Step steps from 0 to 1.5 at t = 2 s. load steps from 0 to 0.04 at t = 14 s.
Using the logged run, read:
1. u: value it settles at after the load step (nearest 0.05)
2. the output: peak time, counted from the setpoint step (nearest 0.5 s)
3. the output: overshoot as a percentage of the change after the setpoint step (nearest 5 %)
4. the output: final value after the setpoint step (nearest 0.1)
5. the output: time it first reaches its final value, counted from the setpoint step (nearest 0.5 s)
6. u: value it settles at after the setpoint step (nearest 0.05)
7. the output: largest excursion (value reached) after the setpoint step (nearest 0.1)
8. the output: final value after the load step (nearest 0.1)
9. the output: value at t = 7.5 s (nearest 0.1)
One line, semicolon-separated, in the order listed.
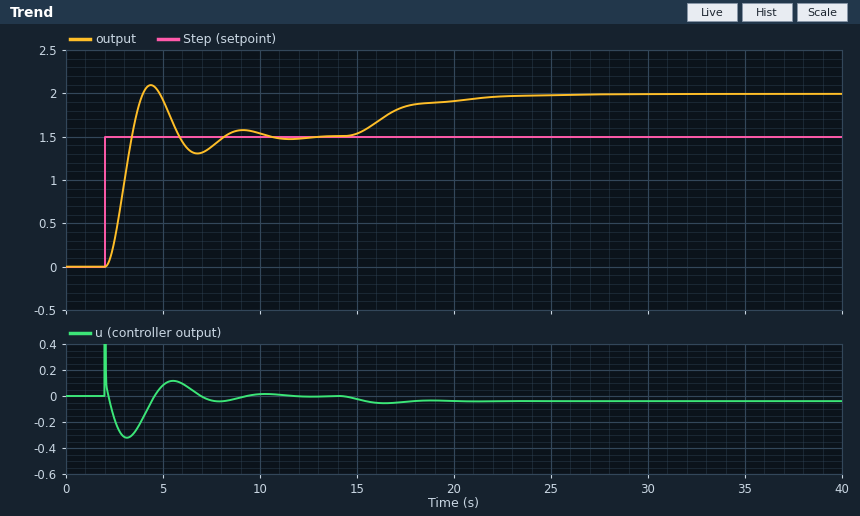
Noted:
-0.05; 2.5 s; 40 %; 1.5; 1.5 s; 0.00; 2.1; 2.0; 1.4
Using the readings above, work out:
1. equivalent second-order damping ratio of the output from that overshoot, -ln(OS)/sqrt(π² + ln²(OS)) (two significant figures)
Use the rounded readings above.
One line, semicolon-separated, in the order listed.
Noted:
0.28
